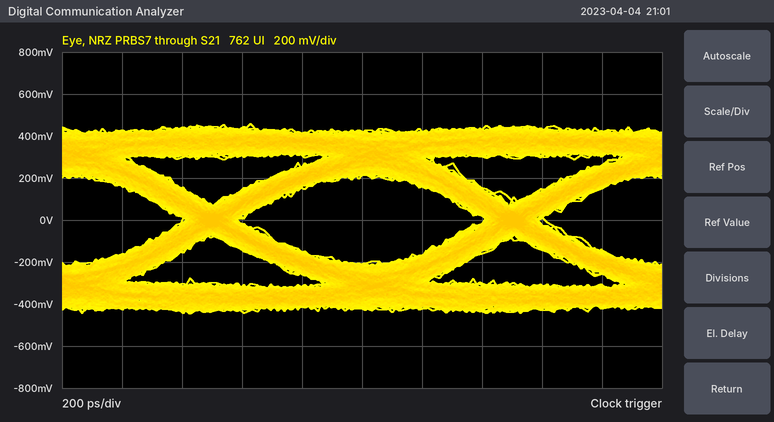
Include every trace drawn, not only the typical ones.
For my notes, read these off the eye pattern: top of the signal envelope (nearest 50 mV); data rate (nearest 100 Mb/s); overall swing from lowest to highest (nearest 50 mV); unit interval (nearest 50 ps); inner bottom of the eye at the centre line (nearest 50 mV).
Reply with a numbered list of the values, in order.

1. 450 mV
2. 1.0 Gb/s
3. 900 mV
4. 1.00 ns
5. -200 mV
